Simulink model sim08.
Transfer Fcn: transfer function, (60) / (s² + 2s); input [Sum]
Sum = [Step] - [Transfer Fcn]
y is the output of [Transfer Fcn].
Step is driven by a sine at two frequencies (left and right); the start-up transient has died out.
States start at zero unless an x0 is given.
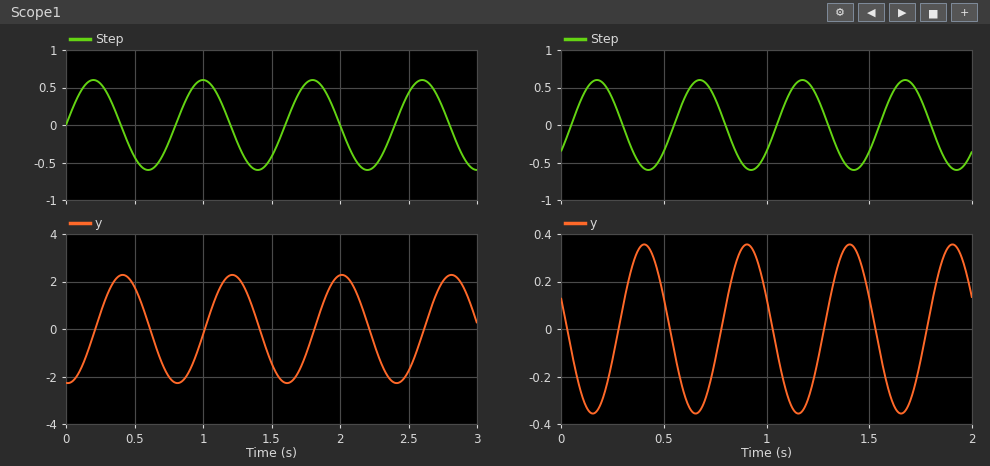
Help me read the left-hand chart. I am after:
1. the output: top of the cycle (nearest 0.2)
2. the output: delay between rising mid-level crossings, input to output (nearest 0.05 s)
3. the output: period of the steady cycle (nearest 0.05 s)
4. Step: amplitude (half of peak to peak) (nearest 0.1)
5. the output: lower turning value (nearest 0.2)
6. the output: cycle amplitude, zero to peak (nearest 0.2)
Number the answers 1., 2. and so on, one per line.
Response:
1. 2.2
2. 0.20 s
3. 0.80 s
4. 0.6
5. -2.2
6. 2.2
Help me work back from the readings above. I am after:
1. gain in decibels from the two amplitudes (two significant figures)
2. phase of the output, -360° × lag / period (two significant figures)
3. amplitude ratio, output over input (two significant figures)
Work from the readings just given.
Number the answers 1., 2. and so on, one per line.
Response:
1. 11 dB
2. -90°
3. 3.7
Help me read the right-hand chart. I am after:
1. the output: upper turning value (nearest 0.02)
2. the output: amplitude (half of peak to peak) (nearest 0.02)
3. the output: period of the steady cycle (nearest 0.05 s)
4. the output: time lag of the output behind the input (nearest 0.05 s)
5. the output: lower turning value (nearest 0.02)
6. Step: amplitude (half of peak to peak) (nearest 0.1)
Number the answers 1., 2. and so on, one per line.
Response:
1. 0.36
2. 0.36
3. 0.50 s
4. 0.25 s
5. -0.36
6. 0.6
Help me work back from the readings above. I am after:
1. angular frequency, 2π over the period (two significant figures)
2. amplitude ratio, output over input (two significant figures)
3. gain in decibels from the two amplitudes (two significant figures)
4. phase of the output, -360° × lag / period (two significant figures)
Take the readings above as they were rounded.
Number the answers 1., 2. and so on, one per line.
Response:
1. 13 rad/s
2. 0.60
3. -4.4 dB
4. -180°
